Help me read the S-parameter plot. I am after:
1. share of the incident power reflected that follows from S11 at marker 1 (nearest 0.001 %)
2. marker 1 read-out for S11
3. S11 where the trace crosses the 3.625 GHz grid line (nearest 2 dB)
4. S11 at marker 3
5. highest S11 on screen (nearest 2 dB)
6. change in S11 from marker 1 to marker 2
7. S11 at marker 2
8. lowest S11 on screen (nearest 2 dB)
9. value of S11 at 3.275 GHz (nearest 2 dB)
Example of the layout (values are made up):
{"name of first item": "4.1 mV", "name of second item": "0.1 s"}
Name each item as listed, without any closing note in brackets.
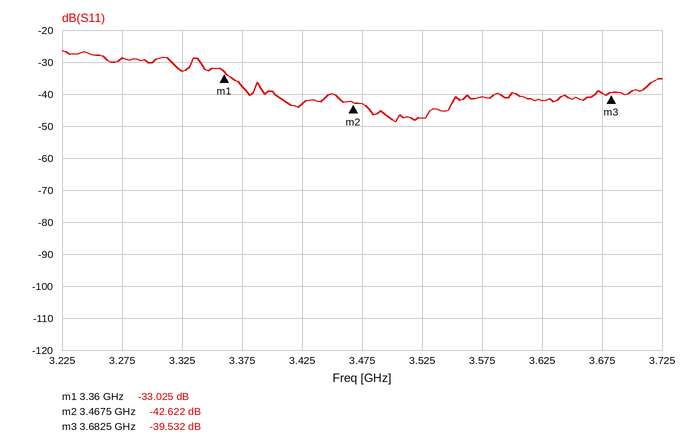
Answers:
{"share of the incident power reflected that follows from S11 at marker 1": "0.050 %", "marker 1 read-out for S11": "-33.025 dB", "S11 where the trace crosses the 3.625 GHz grid line": "-42 dB", "S11 at marker 3": "-39.532 dB", "highest S11 on screen": "-26 dB", "change in S11 from marker 1 to marker 2": "-9.597 dB", "S11 at marker 2": "-42.622 dB", "lowest S11 on screen": "-48 dB", "value of S11 at 3.275 GHz": "-28 dB"}
